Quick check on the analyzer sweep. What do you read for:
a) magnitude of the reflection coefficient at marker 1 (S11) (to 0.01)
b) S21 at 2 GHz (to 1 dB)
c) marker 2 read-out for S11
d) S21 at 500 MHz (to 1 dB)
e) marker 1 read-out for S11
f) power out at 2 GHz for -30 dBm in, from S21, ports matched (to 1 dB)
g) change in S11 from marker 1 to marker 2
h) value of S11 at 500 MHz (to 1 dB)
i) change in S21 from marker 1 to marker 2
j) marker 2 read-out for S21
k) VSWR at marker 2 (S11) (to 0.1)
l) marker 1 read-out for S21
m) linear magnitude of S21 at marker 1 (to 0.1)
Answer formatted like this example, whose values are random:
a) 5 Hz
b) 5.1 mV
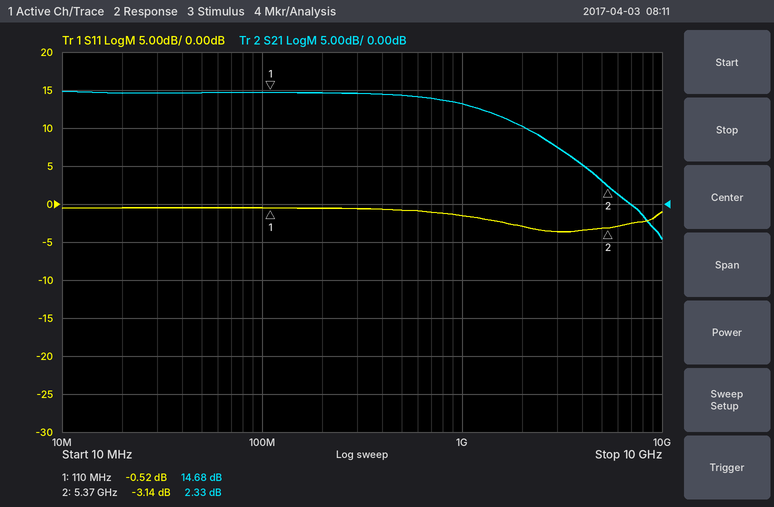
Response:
a) 0.94
b) 10 dB
c) -3.14 dB
d) 14 dB
e) -0.52 dB
f) -20 dBm
g) -2.62 dB
h) -1 dB
i) -12.35 dB
j) 2.33 dB
k) 5.6
l) 14.68 dB
m) 5.4
